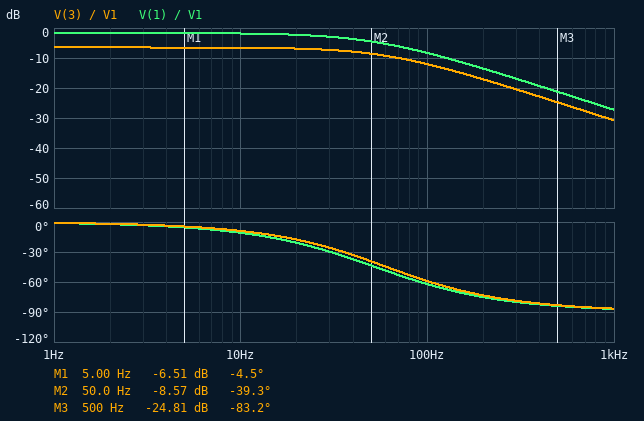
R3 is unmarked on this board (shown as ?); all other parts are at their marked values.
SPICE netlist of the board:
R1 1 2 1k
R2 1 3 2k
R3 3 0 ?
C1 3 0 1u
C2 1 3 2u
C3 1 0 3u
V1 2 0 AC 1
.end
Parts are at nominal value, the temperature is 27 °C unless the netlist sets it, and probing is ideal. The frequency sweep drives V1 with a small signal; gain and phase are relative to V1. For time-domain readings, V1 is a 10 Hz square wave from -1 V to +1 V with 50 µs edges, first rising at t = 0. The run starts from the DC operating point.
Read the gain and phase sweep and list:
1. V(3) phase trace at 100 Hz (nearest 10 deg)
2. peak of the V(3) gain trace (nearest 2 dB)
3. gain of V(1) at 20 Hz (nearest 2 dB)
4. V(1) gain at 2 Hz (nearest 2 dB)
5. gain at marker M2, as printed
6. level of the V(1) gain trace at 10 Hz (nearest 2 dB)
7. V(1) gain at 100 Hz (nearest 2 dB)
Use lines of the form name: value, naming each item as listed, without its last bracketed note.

V(3) phase trace at 100 Hz: -60 deg
peak of the V(3) gain trace: -6 dB
gain of V(1) at 20 Hz: -2 dB
V(1) gain at 2 Hz: -2 dB
gain at marker M2, as printed: -8.57 dB
level of the V(1) gain trace at 10 Hz: -2 dB
V(1) gain at 100 Hz: -8 dB
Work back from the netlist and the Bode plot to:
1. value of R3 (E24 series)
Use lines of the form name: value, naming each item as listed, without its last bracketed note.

value of R3: 2.7 kΩ
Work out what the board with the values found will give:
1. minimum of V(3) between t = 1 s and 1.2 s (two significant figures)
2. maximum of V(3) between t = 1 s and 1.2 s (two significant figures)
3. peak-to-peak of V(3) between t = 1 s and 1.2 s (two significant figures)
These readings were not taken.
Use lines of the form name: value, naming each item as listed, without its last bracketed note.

minimum of V(3) between t = 1 s and 1.2 s: -470 mV
maximum of V(3) between t = 1 s and 1.2 s: 470 mV
peak-to-peak of V(3) between t = 1 s and 1.2 s: 950 mV
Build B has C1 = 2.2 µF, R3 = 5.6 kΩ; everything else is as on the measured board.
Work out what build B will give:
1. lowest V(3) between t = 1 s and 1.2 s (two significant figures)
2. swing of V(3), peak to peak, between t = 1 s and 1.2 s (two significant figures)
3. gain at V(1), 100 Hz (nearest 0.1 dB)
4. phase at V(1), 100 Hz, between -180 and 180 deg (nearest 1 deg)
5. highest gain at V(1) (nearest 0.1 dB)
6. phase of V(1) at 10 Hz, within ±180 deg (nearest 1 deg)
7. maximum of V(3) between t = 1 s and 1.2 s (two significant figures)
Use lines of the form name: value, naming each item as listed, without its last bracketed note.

lowest V(3) between t = 1 s and 1.2 s: -650 mV
swing of V(3), peak to peak, between t = 1 s and 1.2 s: 1.3 V
gain at V(1), 100 Hz: -9.0 dB
phase at V(1), 100 Hz, between -180 and 180 deg: -65 deg
highest gain at V(1): -1.1 dB
phase of V(1) at 10 Hz, within ±180 deg: -13 deg
maximum of V(3) between t = 1 s and 1.2 s: 650 mV
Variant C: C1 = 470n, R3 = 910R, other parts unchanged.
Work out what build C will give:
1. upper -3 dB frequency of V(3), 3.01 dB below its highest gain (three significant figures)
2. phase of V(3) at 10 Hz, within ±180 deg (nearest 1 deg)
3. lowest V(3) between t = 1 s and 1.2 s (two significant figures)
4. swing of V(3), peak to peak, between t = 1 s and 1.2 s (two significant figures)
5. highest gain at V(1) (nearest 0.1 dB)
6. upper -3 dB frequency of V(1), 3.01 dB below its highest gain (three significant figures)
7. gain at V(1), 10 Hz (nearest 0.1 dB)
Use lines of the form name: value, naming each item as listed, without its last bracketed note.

upper -3 dB frequency of V(3), 3.01 dB below its highest gain: 172 Hz
phase of V(3) at 10 Hz, within ±180 deg: -2 deg
lowest V(3) between t = 1 s and 1.2 s: -260 mV
swing of V(3), peak to peak, between t = 1 s and 1.2 s: 510 mV
highest gain at V(1): -2.6 dB
upper -3 dB frequency of V(1), 3.01 dB below its highest gain: 51.8 Hz
gain at V(1), 10 Hz: -2.7 dB
